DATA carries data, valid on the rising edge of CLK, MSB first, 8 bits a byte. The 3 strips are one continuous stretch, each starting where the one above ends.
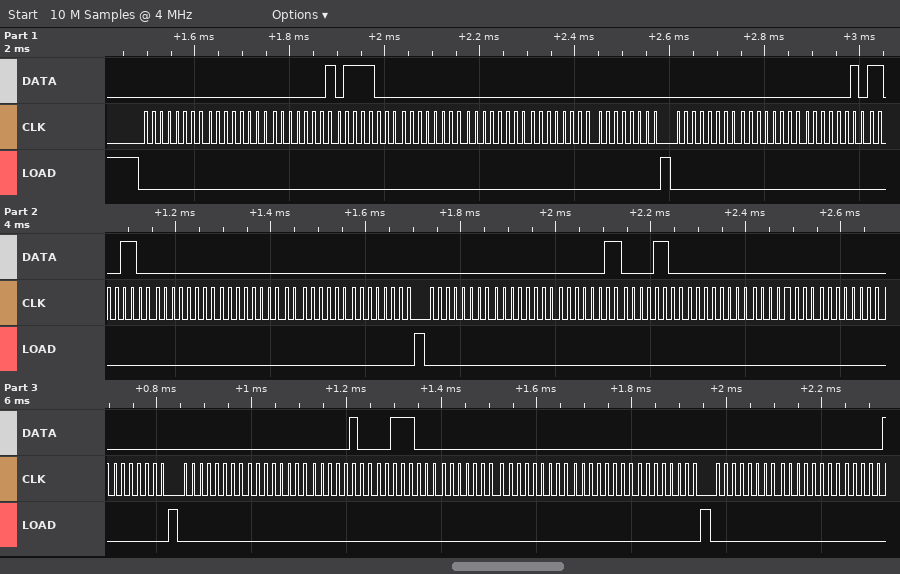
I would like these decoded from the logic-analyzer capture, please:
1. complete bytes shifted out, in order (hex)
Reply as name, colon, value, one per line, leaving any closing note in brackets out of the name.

complete bytes shifted out, in order: 00 00 01 78 00 00 00 00 00 00 02 CC 00 00 00 00 00 00 03 0C 00 00 00 00 00 00 04 38 00 00 00 00 00 00
